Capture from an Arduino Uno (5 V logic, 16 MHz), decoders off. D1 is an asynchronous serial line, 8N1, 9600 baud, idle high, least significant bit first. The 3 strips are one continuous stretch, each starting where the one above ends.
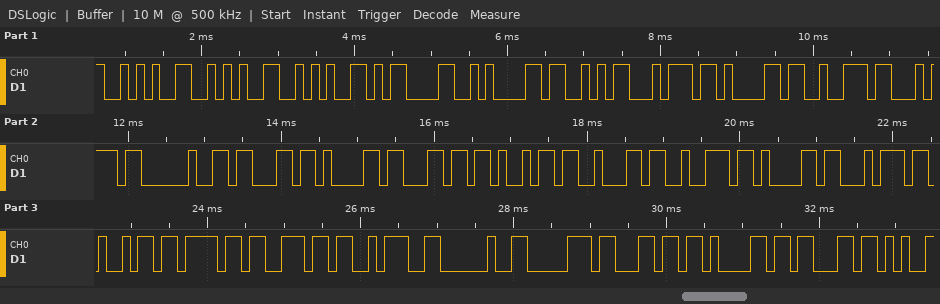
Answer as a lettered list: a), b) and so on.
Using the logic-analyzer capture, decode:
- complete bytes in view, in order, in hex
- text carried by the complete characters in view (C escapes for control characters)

a) 2A 2A 2A 0D 0A 53 74 61 72 74 20 63 61 6C 69 62 72 61 74 69 6F 6E 3A 20 70 6C 61 63
b) "***\r\nStart calibration: plac"
